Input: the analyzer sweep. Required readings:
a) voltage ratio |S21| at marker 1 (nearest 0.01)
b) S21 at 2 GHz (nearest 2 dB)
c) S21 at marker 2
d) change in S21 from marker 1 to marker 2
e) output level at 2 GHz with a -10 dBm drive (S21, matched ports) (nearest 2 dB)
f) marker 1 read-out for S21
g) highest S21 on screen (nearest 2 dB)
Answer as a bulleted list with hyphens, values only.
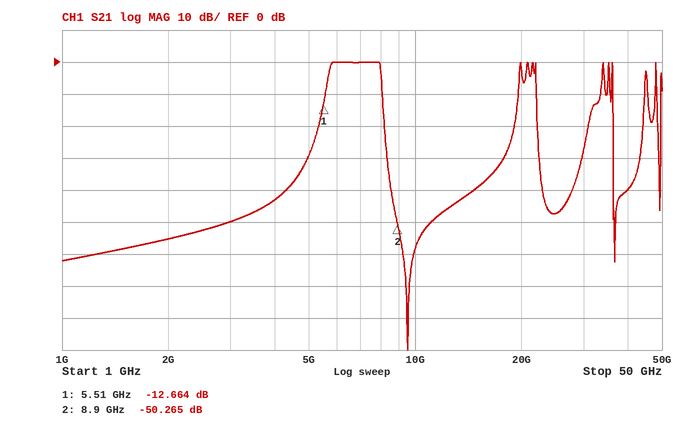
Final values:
- 0.23
- -56 dB
- -50.265 dB
- -37.601 dB
- -66 dBm
- -12.664 dB
- 0 dB
